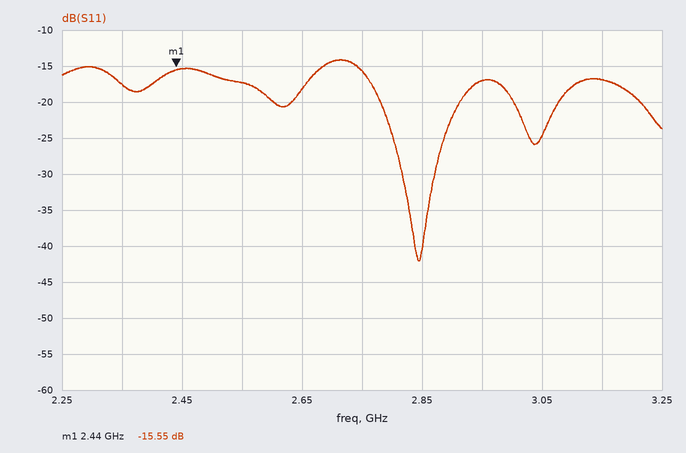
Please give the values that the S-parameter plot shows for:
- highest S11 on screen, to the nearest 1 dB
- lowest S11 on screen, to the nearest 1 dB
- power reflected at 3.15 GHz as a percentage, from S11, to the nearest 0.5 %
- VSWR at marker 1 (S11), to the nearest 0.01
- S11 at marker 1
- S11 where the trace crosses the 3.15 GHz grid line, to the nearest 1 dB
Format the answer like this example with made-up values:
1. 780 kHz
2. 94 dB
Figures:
1. -14 dB
2. -42 dB
3. 2.0 %
4. 1.40
5. -15.55 dB
6. -17 dB
